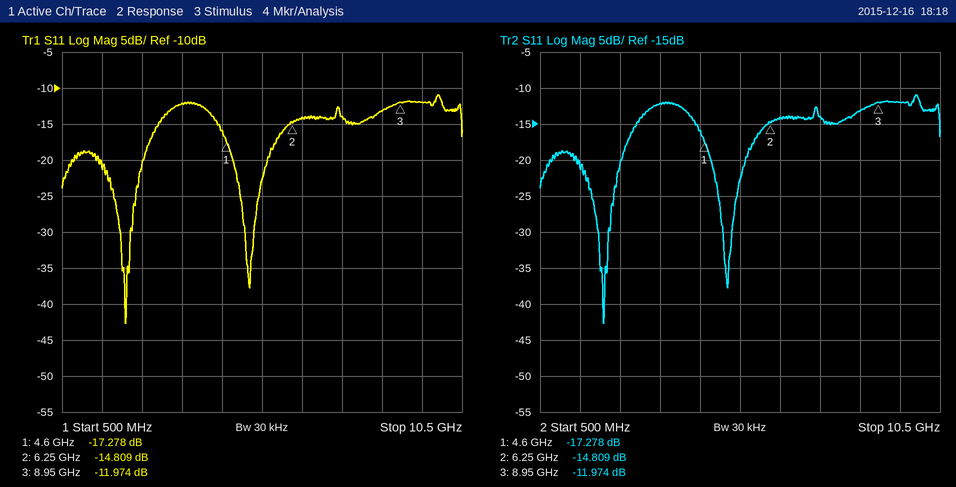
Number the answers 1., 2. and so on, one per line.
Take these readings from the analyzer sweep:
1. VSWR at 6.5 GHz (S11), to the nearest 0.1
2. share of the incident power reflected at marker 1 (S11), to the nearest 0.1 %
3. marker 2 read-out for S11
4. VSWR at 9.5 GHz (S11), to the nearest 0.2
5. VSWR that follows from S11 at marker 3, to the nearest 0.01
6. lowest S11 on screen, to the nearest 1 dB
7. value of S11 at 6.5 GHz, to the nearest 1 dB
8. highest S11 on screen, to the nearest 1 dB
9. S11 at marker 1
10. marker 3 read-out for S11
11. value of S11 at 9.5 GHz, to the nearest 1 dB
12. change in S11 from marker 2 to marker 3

1. 1.5
2. 1.9 %
3. -14.809 dB
4. 1.6
5. 1.67
6. -43 dB
7. -14 dB
8. -11 dB
9. -17.278 dB
10. -11.974 dB
11. -12 dB
12. 2.835 dB
